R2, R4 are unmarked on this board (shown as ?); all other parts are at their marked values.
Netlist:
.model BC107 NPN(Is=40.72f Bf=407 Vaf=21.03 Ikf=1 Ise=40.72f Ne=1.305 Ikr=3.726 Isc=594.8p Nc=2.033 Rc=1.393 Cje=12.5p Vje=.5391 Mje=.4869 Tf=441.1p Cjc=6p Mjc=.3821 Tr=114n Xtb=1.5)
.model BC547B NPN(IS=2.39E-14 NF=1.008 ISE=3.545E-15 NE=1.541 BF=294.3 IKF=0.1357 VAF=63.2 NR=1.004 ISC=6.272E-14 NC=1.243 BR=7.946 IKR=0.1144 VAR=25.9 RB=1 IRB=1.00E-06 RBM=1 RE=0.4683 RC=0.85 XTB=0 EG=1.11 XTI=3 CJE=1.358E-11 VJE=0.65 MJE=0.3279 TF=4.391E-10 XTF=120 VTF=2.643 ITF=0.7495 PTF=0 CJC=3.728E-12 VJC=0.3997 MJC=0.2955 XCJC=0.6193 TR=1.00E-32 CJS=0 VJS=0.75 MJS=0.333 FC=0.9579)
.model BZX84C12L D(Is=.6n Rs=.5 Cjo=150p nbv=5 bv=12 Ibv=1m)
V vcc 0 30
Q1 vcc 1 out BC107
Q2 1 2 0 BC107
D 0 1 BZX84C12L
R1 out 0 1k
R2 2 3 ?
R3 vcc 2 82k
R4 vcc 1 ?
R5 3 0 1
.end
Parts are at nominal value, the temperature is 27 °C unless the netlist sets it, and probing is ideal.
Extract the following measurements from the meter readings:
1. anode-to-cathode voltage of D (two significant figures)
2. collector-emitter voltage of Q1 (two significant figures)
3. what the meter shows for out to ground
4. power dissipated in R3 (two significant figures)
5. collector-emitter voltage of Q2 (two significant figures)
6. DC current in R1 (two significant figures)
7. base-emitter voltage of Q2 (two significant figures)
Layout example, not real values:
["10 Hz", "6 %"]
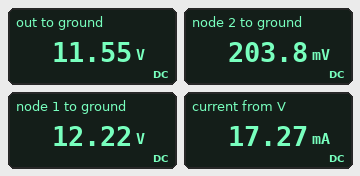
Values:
["-12 V", "18 V", "11.55 V", "11 mW", "12 V", "12 mA", "200 mV"]
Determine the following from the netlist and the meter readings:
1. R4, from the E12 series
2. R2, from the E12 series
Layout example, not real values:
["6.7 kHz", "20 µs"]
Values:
["3.3 kΩ", "560 Ω"]
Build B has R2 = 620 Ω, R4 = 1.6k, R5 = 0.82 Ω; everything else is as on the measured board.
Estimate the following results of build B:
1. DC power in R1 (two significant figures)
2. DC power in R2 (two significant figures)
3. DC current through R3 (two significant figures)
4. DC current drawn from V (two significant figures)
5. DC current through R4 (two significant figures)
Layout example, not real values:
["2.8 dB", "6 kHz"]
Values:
["140 mW", "82 µW", "360 µA", "23 mA", "11 mA"]
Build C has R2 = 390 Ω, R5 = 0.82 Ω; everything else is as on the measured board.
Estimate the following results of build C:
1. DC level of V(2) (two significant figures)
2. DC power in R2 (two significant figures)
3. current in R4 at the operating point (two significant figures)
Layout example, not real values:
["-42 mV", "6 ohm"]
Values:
["140 mV", "52 µW", "5.4 mA"]
